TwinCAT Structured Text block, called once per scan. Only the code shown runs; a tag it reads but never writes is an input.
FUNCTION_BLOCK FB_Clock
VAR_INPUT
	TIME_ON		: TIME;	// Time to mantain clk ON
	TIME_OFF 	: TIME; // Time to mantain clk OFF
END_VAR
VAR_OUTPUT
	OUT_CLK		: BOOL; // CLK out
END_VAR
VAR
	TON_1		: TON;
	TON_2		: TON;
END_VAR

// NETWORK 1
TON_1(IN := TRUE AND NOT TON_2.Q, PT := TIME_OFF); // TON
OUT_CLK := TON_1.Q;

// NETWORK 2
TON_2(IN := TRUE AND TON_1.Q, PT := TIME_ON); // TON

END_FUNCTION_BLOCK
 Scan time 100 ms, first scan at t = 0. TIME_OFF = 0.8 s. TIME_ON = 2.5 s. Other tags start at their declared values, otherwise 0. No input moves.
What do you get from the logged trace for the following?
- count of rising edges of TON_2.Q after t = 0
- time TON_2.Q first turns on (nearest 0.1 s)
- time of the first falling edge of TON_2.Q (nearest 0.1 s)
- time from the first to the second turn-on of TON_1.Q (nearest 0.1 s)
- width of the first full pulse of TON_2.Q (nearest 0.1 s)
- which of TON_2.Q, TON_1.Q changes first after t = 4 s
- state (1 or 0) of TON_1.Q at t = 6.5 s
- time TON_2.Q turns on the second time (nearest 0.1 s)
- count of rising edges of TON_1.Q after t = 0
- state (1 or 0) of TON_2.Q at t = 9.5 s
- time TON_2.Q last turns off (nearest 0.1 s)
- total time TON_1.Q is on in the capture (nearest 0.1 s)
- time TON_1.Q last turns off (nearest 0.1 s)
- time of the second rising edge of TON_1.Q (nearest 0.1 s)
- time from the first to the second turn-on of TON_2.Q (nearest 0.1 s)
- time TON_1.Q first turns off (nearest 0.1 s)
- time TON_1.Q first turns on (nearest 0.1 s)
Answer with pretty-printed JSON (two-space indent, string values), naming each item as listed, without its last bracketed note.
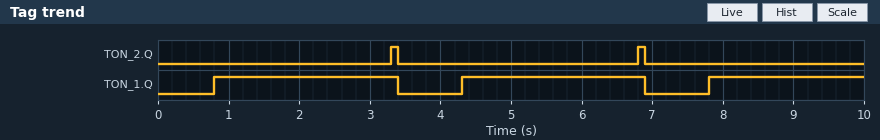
{
  "count of rising edges of TON_2.Q after t = 0": "2",
  "time TON_2.Q first turns on": "3.3 s",
  "time of the first falling edge of TON_2.Q": "3.4 s",
  "time from the first to the second turn-on of TON_1.Q": "3.5 s",
  "width of the first full pulse of TON_2.Q": "0.1 s",
  "which of TON_2.Q, TON_1.Q changes first after t = 4 s": "TON_1.Q",
  "state (1 or 0) of TON_1.Q at t = 6.5 s": "1",
  "time TON_2.Q turns on the second time": "6.8 s",
  "count of rising edges of TON_1.Q after t = 0": "3",
  "state (1 or 0) of TON_2.Q at t = 9.5 s": "0",
  "time TON_2.Q last turns off": "6.9 s",
  "total time TON_1.Q is on in the capture": "7.4 s",
  "time TON_1.Q last turns off": "6.9 s",
  "time of the second rising edge of TON_1.Q": "4.3 s",
  "time from the first to the second turn-on of TON_2.Q": "3.5 s",
  "time TON_1.Q first turns off": "3.4 s",
  "time TON_1.Q first turns on": "0.8 s"
}
